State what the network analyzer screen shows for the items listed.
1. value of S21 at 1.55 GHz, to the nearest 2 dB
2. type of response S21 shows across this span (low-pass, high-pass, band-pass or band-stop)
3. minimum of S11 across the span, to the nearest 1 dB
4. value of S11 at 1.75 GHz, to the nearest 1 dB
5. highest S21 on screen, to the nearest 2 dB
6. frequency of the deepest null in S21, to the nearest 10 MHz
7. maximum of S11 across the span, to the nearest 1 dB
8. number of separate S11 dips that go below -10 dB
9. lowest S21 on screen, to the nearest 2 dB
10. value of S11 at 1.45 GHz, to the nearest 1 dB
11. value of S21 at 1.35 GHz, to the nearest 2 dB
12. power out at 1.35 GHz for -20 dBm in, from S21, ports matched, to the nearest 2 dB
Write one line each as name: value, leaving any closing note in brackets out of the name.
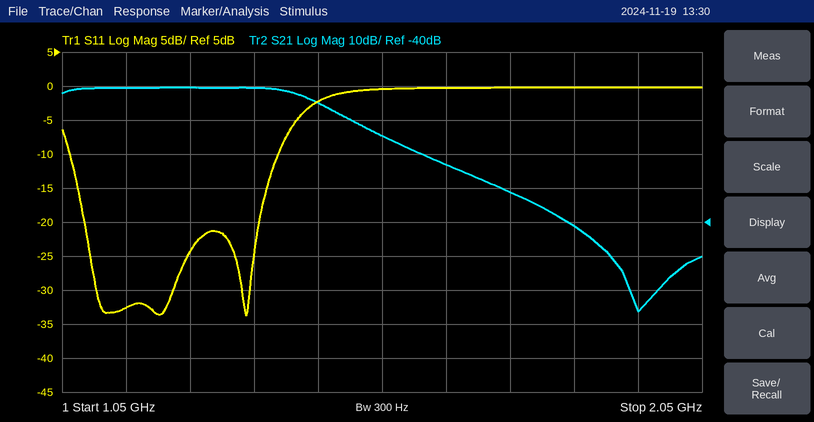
value of S21 at 1.55 GHz, to the nearest 2 dB: -14 dB
type of response S21 shows across this span: low-pass
minimum of S11 across the span, to the nearest 1 dB: -34 dB
value of S11 at 1.75 GHz, to the nearest 1 dB: 0 dB
highest S21 on screen, to the nearest 2 dB: 0 dB
frequency of the deepest null in S21, to the nearest 10 MHz: 1.95 GHz
maximum of S11 across the span, to the nearest 1 dB: 0 dB
number of separate S11 dips that go below -10 dB: 2
lowest S21 on screen, to the nearest 2 dB: -66 dB
value of S11 at 1.45 GHz, to the nearest 1 dB: -2 dB
value of S21 at 1.35 GHz, to the nearest 2 dB: 0 dB
power out at 1.35 GHz for -20 dBm in, from S21, ports matched, to the nearest 2 dB: -20 dBm
